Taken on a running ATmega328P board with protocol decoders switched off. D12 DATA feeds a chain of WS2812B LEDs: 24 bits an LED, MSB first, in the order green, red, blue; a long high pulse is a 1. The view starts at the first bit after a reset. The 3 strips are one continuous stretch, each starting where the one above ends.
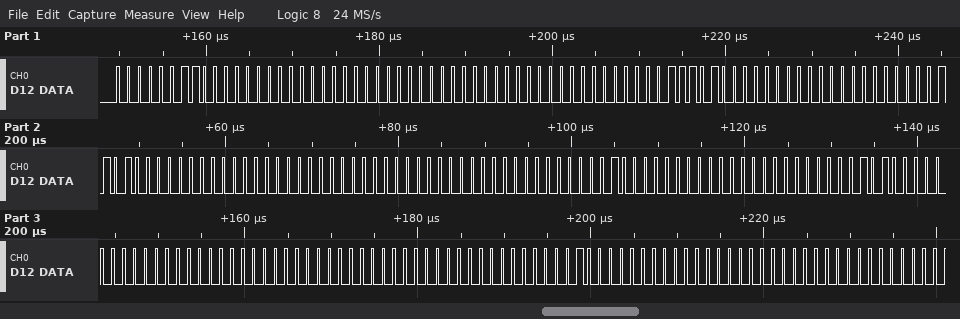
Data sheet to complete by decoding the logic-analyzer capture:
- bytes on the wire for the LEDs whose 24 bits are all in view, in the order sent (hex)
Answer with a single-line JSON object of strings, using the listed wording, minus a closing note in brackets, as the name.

{"bytes on the wire for the LEDs whose 24 bits are all in view, in the order sent": "03 00 00 00 00 00 1D 00 00 0D 00 00 00 00 00 08 00 00 14 00 00 00 00 00 01 00 00"}
